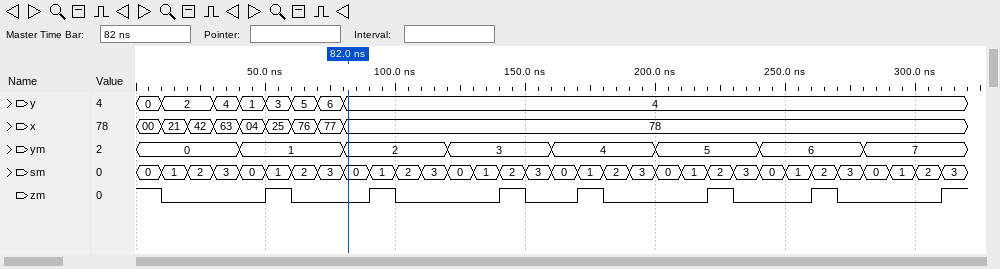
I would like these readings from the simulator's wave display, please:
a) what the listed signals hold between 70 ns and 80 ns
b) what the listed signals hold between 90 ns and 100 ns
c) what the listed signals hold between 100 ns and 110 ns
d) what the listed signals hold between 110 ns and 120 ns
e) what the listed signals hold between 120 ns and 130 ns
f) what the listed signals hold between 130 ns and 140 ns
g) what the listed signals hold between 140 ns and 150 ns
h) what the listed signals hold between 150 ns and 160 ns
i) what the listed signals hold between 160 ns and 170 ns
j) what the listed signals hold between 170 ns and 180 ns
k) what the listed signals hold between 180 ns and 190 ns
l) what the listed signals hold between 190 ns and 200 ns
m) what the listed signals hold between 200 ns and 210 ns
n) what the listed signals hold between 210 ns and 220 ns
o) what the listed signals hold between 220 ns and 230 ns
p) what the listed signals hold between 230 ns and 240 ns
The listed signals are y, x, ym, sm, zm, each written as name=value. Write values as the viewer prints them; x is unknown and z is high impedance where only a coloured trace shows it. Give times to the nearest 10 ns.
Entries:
y=6, x=77, ym=1, sm=3, zm=0
y=4, x=78, ym=2, sm=1, zm=1
y=4, x=78, ym=2, sm=2, zm=0
y=4, x=78, ym=2, sm=3, zm=0
y=4, x=78, ym=3, sm=0, zm=0
y=4, x=78, ym=3, sm=1, zm=0
y=4, x=78, ym=3, sm=2, zm=1
y=4, x=78, ym=3, sm=3, zm=0
y=4, x=78, ym=4, sm=0, zm=0
y=4, x=78, ym=4, sm=1, zm=1
y=4, x=78, ym=4, sm=2, zm=0
y=4, x=78, ym=4, sm=3, zm=0
y=4, x=78, ym=5, sm=0, zm=0
y=4, x=78, ym=5, sm=1, zm=0
y=4, x=78, ym=5, sm=2, zm=1
y=4, x=78, ym=5, sm=3, zm=0
